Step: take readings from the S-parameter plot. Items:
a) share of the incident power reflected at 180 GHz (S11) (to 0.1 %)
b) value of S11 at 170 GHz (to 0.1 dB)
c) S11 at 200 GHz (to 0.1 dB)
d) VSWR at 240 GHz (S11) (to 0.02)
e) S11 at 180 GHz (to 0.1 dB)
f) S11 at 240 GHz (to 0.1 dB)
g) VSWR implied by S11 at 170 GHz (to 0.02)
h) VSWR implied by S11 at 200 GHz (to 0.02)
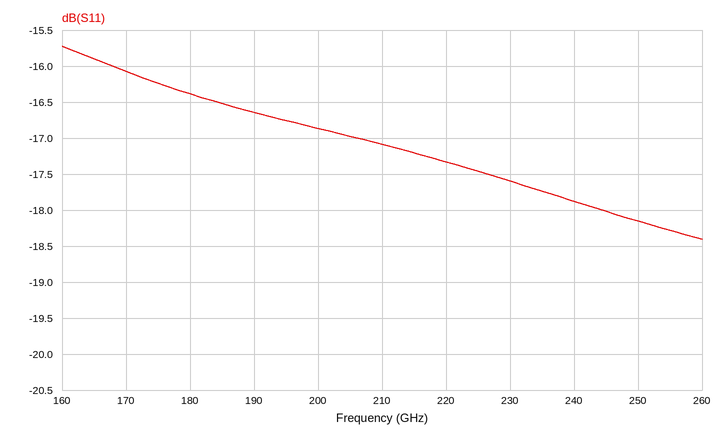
2.3 %
-16.1 dB
-16.9 dB
1.30
-16.4 dB
-17.9 dB
1.38
1.34
